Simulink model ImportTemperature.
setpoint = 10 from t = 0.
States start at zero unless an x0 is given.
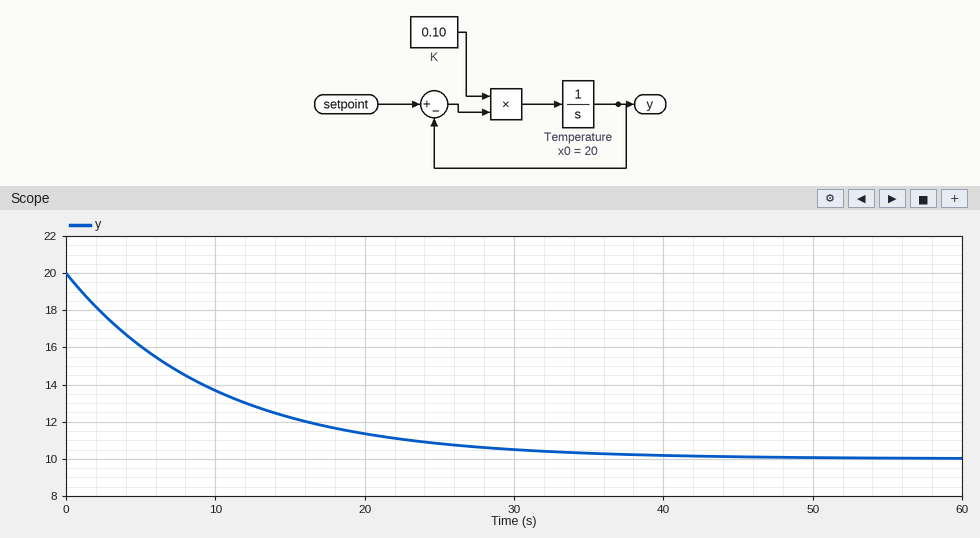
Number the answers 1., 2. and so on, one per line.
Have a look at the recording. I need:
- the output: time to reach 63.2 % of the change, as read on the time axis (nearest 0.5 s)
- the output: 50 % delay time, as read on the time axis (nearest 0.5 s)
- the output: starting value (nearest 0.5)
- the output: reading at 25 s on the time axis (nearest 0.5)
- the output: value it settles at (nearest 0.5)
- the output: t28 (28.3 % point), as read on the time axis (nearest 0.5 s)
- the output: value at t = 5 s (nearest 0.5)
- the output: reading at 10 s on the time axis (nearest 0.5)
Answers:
1. 10.0 s
2. 7.0 s
3. 20.0
4. 11.0
5. 10.0
6. 3.5 s
7. 16.0
8. 13.5
